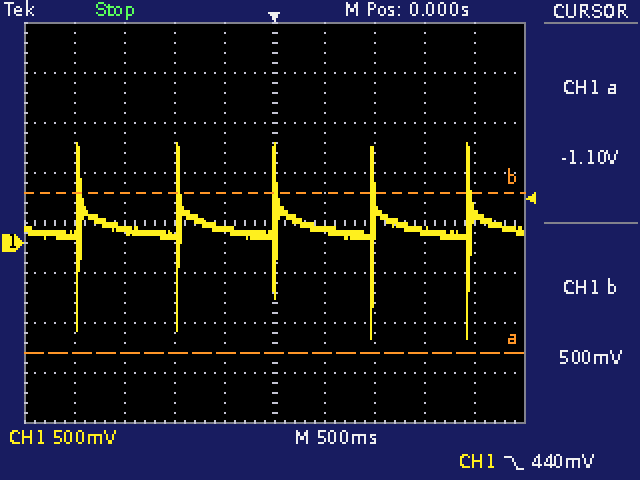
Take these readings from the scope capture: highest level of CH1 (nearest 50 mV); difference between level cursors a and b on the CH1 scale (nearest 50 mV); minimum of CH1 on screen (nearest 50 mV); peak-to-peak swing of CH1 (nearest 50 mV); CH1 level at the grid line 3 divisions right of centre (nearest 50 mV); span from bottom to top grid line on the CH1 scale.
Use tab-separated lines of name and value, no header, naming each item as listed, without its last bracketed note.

highest level of CH1	1.00 V
difference between level cursors a and b on the CH1 scale	1.60 V
minimum of CH1 on screen	-950 mV
peak-to-peak swing of CH1	1.95 V
CH1 level at the grid line 3 divisions right of centre	100 mV
span from bottom to top grid line on the CH1 scale	4 V
